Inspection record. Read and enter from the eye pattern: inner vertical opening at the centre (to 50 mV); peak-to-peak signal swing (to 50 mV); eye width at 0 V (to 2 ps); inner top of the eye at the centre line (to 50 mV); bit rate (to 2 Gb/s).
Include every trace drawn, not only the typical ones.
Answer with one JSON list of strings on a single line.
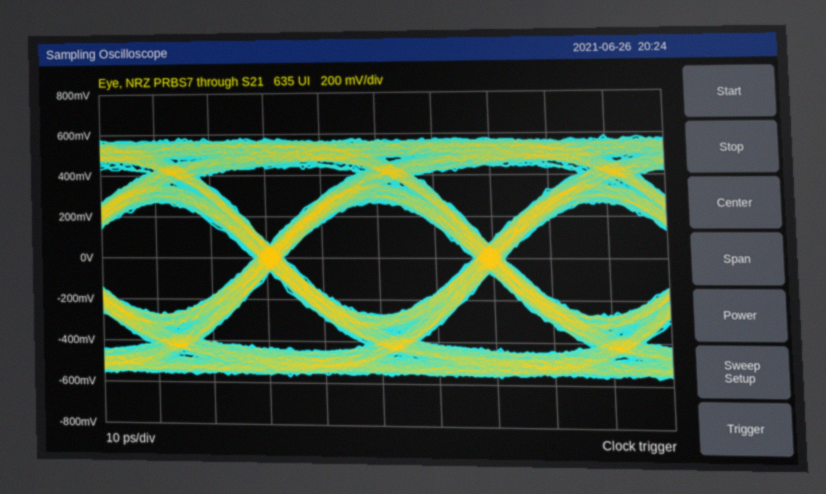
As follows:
["550 mV", "1.15 V", "34 ps", "250 mV", "26 Gb/s"]
